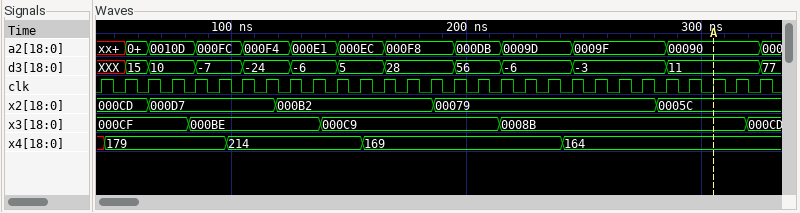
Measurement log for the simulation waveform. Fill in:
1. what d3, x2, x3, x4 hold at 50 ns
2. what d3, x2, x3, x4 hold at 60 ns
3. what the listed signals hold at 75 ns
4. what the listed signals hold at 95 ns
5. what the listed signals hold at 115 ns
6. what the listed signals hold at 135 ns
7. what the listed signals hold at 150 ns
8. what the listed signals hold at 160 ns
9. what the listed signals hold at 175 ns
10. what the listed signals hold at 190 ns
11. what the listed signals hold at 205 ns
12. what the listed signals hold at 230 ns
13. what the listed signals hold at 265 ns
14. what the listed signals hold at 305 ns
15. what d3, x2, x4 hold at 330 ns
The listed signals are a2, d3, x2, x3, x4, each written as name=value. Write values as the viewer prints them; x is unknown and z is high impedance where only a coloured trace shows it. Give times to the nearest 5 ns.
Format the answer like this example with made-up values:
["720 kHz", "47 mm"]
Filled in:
["d3=XXX, x2=000CD, x3=000CF, x4=179", "d3=15, x2=000CD, x3=000CF, x4=179", "a2=0010D, d3=10, x2=000D7, x3=000CF, x4=179", "a2=000FC, d3=-7, x2=000D7, x3=000BE, x4=179", "a2=000F4, d3=-24, x2=000D7, x3=000BE, x4=214", "a2=000E1, d3=-6, x2=000B2, x3=000BE, x4=214", "a2=000EC, d3=5, x2=000B2, x3=000C9, x4=214", "a2=000EC, d3=5, x2=000B2, x3=000C9, x4=169", "a2=000F8, d3=28, x2=000B2, x3=000C9, x4=169", "a2=000F8, d3=28, x2=00079, x3=000C9, x4=169", "a2=000DB, d3=56, x2=00079, x3=000C9, x4=169", "a2=0009D, d3=-6, x2=00079, x3=0008B, x4=169", "a2=0009F, d3=-3, x2=00079, x3=0008B, x4=164", "a2=00090, d3=11, x2=0005C, x3=0008B, x4=164", "d3=77, x2=0005C, x4=164"]
